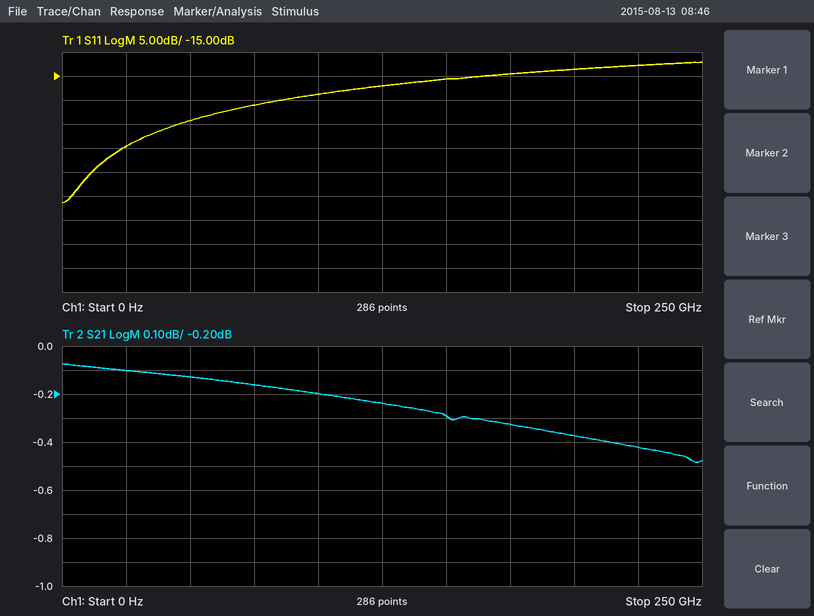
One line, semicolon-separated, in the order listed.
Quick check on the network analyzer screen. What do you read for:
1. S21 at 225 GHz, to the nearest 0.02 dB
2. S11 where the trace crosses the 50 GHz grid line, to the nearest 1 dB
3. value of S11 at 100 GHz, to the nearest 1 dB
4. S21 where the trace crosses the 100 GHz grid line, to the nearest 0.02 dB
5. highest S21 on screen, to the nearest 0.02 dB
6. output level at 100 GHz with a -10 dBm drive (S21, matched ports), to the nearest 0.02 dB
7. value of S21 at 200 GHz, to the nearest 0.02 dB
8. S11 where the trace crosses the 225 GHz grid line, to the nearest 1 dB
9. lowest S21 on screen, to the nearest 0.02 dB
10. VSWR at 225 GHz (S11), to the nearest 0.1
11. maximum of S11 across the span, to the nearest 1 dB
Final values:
-0.42 dB; -24 dB; -19 dB; -0.20 dB; -0.08 dB; -10.20 dBm; -0.38 dB; -13 dB; -0.48 dB; 1.6; -12 dB
